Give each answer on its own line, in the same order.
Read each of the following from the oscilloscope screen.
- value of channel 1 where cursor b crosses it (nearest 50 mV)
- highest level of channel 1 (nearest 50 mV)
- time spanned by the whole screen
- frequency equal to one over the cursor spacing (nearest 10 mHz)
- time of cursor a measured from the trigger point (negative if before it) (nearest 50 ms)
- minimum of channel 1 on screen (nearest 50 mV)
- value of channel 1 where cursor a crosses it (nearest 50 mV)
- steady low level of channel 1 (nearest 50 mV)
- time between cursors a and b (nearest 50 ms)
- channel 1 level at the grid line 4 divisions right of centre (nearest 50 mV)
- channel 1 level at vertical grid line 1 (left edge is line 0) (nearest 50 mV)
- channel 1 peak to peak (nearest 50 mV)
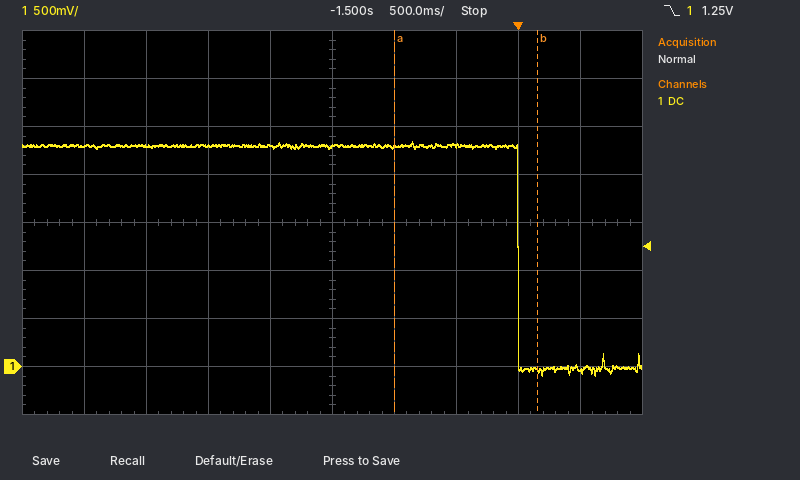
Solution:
-50 mV
2.35 V
5 s
870 mHz
-1.00 s
-100 mV
2.30 V
0 mV
1.15 s
-50 mV
2.30 V
2.45 V
